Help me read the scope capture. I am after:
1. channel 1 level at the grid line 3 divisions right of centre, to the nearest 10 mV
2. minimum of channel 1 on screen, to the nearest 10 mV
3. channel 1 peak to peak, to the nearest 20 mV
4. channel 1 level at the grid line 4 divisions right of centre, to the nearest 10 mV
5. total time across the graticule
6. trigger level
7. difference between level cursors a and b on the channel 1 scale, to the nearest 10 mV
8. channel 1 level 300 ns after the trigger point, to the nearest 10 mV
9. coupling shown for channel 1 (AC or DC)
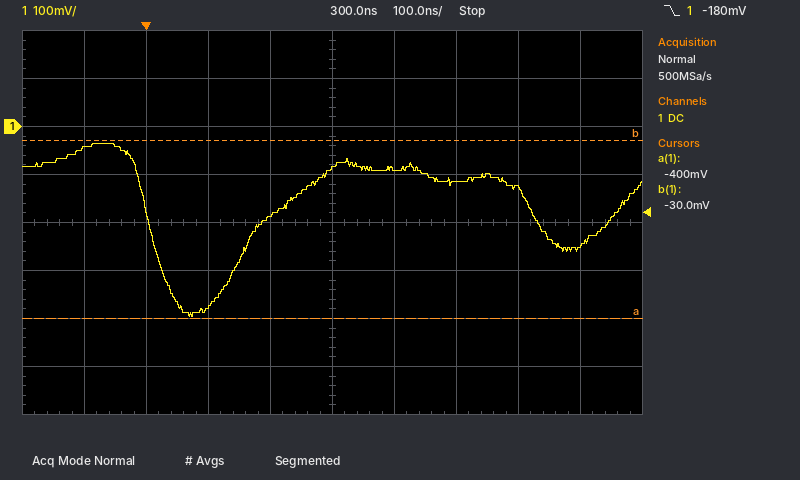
-130 mV
-400 mV
360 mV
-250 mV
1 µs
-180 mV
370 mV
-90 mV
DC
